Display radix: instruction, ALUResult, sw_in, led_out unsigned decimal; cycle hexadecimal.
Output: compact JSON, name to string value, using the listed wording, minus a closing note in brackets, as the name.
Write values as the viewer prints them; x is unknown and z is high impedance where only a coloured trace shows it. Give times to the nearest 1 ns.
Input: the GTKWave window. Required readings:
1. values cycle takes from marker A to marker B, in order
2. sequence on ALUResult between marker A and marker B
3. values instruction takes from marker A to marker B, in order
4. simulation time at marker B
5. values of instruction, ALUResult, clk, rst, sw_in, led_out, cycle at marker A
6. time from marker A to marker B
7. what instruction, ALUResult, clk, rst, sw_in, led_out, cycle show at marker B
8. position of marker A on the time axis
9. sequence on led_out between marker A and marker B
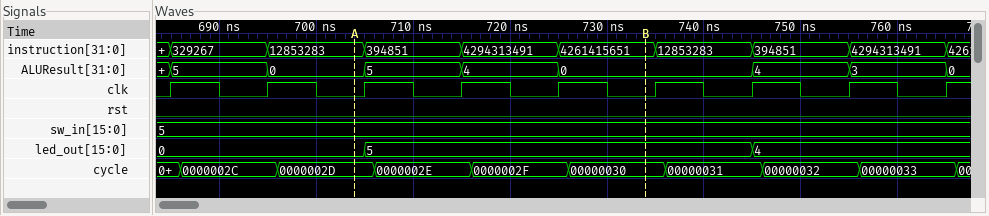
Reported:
{"values cycle takes from marker A to marker B, in order": "0000002D, 0000002E, 0000002F, 00000030", "sequence on ALUResult between marker A and marker B": "0, 5, 4, 0", "values instruction takes from marker A to marker B, in order": "12853283, 394851, 4294313491, 4261415651", "simulation time at marker B": "734 ns", "values of instruction, ALUResult, clk, rst, sw_in, led_out, cycle at marker A": "instruction=12853283, ALUResult=0, clk=0, rst=0, sw_in=5, led_out=0, cycle=0000002D", "time from marker A to marker B": "30 ns", "what instruction, ALUResult, clk, rst, sw_in, led_out, cycle show at marker B": "instruction=4261415651, ALUResult=0, clk=0, rst=0, sw_in=5, led_out=5, cycle=00000030", "position of marker A on the time axis": "704 ns", "sequence on led_out between marker A and marker B": "0, 5"}
